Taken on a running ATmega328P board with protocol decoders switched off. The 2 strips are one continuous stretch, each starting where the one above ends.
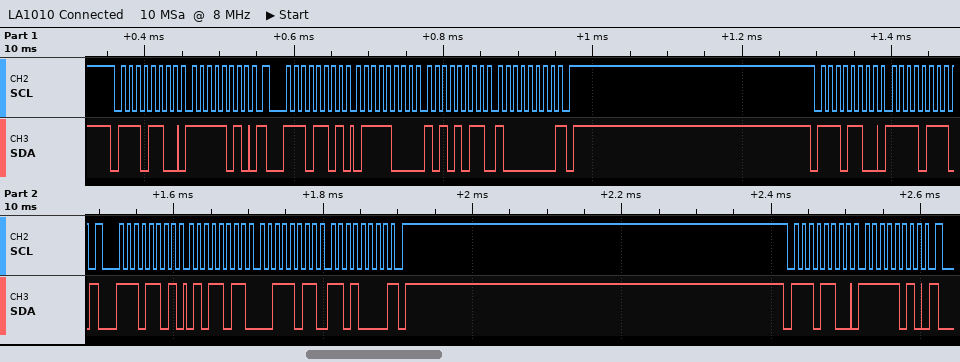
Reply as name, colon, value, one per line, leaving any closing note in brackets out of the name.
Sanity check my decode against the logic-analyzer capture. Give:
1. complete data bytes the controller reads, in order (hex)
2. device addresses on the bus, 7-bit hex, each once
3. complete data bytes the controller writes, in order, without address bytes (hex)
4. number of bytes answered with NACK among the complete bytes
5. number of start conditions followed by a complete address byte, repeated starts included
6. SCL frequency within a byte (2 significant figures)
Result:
complete data bytes the controller reads, in order: 78 AB 80 5B 3B D0
device addresses on the bus, 7-bit hex, each once: 0x76
complete data bytes the controller writes, in order, without address bytes: FA F7 FA
number of bytes answered with NACK among the complete bytes: 2
number of start conditions followed by a complete address byte, repeated starts included: 5
SCL frequency within a byte: 100 kHz
